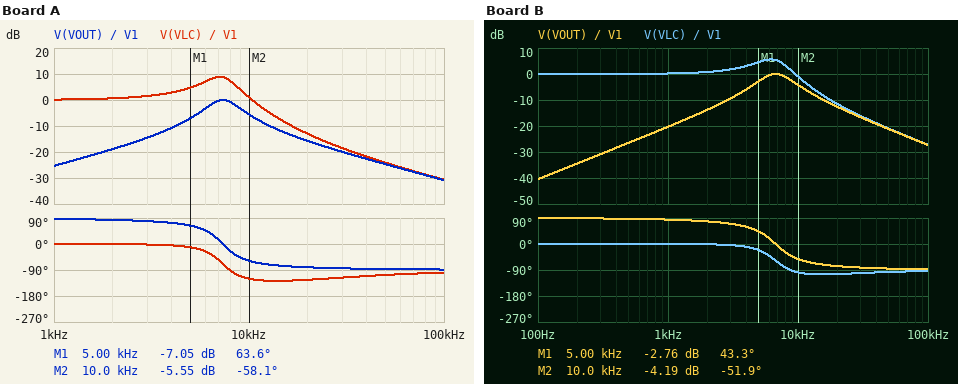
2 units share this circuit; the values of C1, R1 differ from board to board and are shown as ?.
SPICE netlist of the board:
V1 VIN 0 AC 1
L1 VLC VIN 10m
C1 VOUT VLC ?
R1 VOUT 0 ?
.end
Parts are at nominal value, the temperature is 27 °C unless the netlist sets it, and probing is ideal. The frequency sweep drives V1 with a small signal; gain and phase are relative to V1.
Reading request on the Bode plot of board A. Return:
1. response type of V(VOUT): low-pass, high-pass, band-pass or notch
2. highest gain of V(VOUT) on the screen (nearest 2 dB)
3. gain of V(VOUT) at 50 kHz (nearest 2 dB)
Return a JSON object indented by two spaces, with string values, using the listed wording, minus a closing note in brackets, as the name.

{
  "response type of V(VOUT): low-pass, high-pass, band-pass or notch": "band-pass",
  "highest gain of V(VOUT) on the screen": "0 dB",
  "gain of V(VOUT) at 50 kHz": "-24 dB"
}
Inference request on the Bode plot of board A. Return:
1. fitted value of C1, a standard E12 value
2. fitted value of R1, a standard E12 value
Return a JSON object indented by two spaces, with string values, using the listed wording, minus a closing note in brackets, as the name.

{
  "fitted value of C1, a standard E12 value": "47 nF",
  "fitted value of R1, a standard E12 value": "180 Ω"
}
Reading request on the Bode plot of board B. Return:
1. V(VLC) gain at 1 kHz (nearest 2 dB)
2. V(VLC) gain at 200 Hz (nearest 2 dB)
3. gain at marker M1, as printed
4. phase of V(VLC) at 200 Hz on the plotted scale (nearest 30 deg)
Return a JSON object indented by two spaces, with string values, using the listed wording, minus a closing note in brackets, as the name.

{
  "V(VLC) gain at 1 kHz": "0 dB",
  "V(VLC) gain at 200 Hz": "0 dB",
  "gain at marker M1, as printed": "-2.76 dB",
  "phase of V(VLC) at 200 Hz on the plotted scale": "0 deg"
}
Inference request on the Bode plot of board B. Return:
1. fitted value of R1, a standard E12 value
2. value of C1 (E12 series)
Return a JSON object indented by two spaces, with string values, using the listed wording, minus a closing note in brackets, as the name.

{
  "fitted value of R1, a standard E12 value": "270 Ω",
  "value of C1": "56 nF"
}
